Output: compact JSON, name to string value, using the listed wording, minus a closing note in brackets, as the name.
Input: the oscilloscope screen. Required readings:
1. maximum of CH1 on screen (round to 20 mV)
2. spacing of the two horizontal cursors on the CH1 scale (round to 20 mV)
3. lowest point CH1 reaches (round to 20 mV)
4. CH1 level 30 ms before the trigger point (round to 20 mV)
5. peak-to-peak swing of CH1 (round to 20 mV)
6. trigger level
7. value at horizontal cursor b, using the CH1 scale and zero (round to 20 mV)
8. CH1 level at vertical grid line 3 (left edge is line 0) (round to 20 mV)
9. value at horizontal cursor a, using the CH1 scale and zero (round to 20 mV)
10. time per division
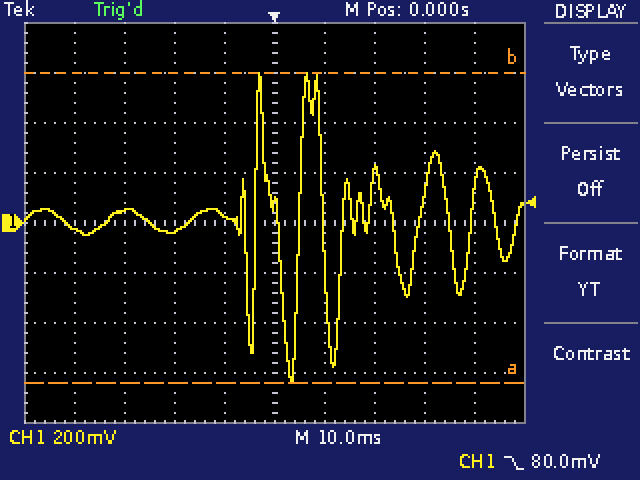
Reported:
{"maximum of CH1 on screen": "600 mV", "spacing of the two horizontal cursors on the CH1 scale": "1.24 V", "lowest point CH1 reaches": "-640 mV", "CH1 level 30 ms before the trigger point": "40 mV", "peak-to-peak swing of CH1": "1.24 V", "trigger level": "80.0 mV", "value at horizontal cursor b, using the CH1 scale and zero": "600 mV", "CH1 level at vertical grid line 3 (left edge is line 0)": "-40 mV", "value at horizontal cursor a, using the CH1 scale and zero": "-640 mV", "time per division": "10 ms"}
